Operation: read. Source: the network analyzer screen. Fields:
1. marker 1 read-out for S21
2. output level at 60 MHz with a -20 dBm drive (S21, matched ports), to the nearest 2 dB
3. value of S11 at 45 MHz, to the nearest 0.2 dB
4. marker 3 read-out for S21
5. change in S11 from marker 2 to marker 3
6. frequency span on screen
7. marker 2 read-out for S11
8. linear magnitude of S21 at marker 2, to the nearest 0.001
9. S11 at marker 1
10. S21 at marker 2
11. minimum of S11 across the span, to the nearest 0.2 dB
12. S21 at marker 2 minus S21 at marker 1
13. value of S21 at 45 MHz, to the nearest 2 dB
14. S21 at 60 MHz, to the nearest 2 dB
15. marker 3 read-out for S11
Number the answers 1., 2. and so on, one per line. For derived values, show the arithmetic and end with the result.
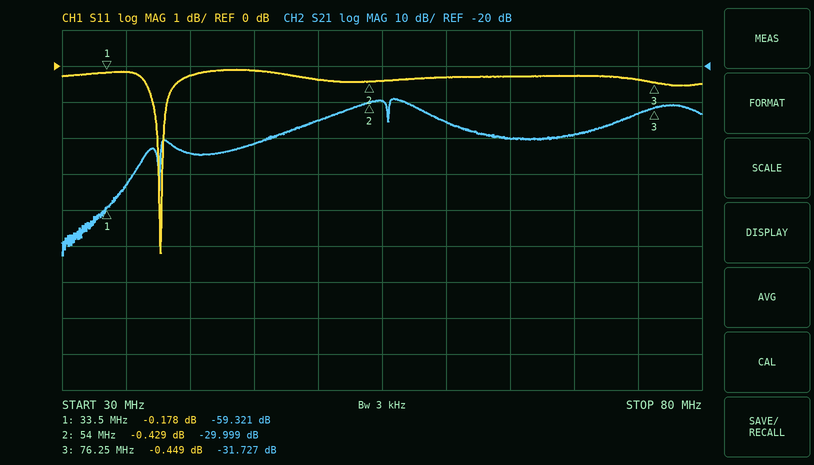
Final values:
1. -59.321 dB
2. -20 dBm + (-36 dB) = -56 dBm
3. -0.2 dB
4. -31.727 dB
5. -0.449 − (-0.429) = -0.020 dB
6. 50 MHz
7. -0.429 dB
8. 10^(-29.999/20) ≈ 0.032
9. -0.178 dB
10. -29.999 dB
11. -5.2 dB
12. -29.999 − (-59.321) = 29.322 dB
13. -42 dB
14. -36 dB
15. -0.449 dB
